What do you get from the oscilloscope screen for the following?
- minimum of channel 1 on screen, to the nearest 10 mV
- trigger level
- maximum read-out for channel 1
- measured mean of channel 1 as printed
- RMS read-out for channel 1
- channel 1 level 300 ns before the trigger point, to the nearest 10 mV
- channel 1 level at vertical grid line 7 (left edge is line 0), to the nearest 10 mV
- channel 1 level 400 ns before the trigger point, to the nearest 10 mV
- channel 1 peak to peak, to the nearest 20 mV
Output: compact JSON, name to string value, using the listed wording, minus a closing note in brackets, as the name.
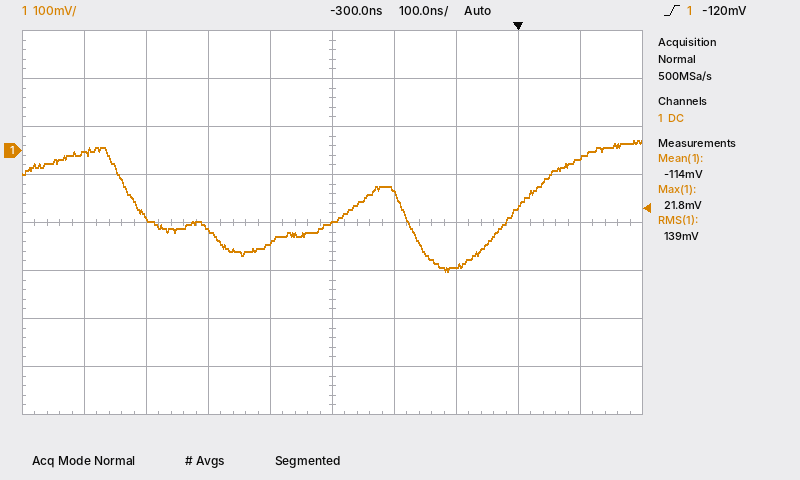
{"minimum of channel 1 on screen, to the nearest 10 mV": "-250 mV", "trigger level": "-120 mV", "maximum read-out for channel 1": "21.8 mV", "measured mean of channel 1 as printed": "-114 mV", "RMS read-out for channel 1": "139 mV", "channel 1 level 300 ns before the trigger point, to the nearest 10 mV": "-150 mV", "channel 1 level at vertical grid line 7 (left edge is line 0), to the nearest 10 mV": "-240 mV", "channel 1 level 400 ns before the trigger point, to the nearest 10 mV": "-190 mV", "channel 1 peak to peak, to the nearest 20 mV": "280 mV"}
